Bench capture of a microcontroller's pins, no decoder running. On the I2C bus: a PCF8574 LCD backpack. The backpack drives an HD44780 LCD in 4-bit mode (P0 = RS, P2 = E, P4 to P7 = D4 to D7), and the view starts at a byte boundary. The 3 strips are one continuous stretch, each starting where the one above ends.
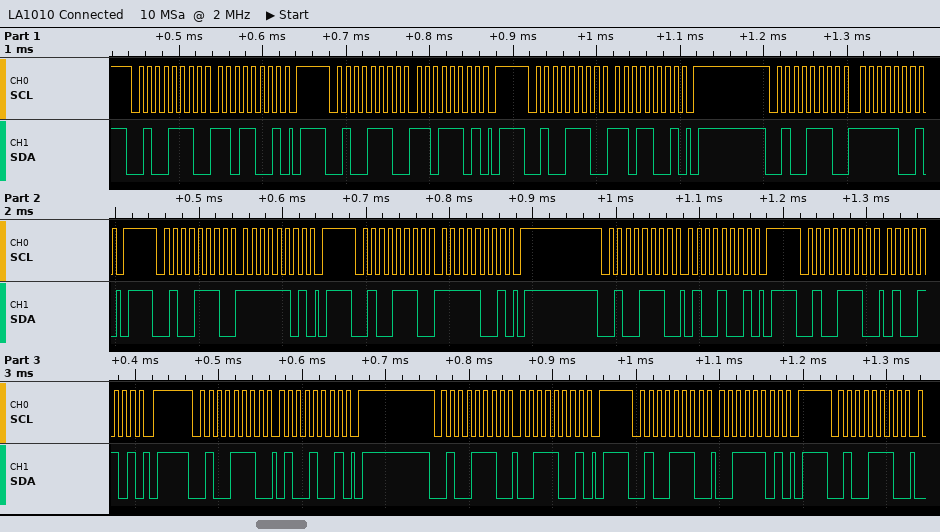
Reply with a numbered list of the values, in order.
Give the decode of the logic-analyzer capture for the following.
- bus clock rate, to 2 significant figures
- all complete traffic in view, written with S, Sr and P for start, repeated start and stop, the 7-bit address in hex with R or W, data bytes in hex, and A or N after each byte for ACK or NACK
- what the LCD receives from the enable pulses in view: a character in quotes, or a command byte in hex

1. 100 kHz
2. S 27W A D9 A P S 27W A DD A P S 27W A D9 A P S 27W A F9 A P S 27W A FD A P S 27W A F9 A P S 27W A 49 A P S 27W A 4D A P S 27W A 49 A P S 27W A 39 A P S 27W A 3D A P S 27W A
3. data 0xDF
